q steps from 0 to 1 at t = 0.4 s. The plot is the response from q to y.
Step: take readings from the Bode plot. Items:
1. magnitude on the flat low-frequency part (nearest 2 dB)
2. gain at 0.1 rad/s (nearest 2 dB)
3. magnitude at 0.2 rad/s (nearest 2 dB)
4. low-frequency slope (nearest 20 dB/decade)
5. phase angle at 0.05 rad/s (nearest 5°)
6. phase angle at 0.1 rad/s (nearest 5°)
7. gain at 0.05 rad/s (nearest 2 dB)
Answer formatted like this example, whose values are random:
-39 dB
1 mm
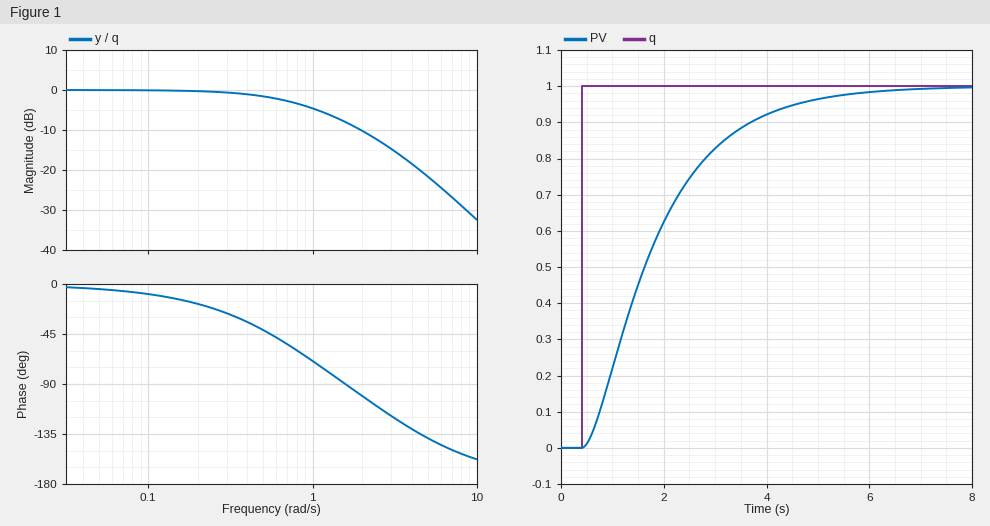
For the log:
0 dB
0 dB
0 dB
0 dB/decade
-5°
-10°
0 dB
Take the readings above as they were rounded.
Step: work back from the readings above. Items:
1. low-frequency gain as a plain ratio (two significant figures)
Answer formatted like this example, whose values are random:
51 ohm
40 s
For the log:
1.0
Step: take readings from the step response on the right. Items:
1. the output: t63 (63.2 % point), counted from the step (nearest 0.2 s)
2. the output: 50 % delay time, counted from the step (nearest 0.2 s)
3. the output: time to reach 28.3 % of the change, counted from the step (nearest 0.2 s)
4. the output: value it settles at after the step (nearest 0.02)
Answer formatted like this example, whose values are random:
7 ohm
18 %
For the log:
1.6 s
1.2 s
0.8 s
1.00
